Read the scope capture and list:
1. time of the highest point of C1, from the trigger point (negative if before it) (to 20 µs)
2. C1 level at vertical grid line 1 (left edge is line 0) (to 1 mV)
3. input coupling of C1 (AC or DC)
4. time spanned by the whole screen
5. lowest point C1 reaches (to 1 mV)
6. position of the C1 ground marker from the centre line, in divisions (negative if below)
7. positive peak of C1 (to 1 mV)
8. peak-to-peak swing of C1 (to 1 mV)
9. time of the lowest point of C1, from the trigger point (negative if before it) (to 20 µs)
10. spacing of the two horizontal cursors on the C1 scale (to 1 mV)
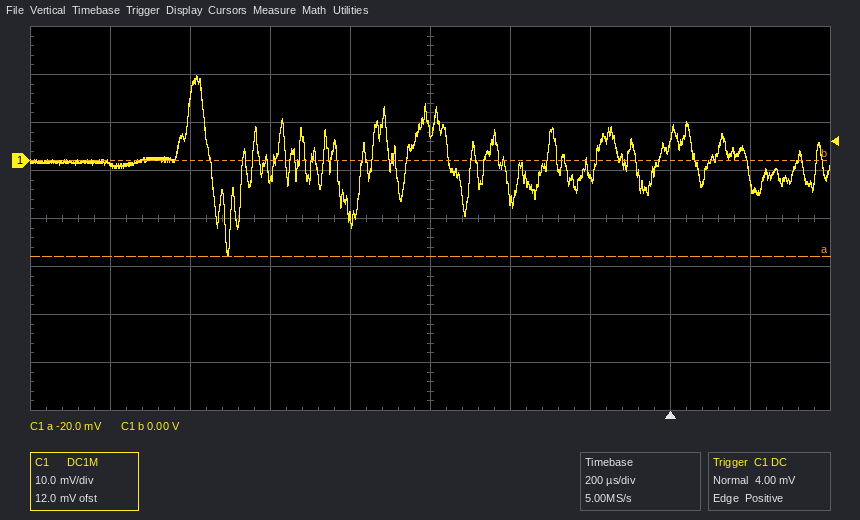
-1.18 ms
-1 mV
DC
2 ms
-20 mV
+1.2 div
18 mV
38 mV
-1.10 ms
20 mV
